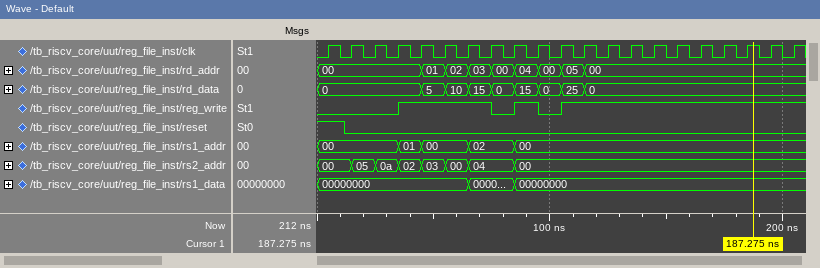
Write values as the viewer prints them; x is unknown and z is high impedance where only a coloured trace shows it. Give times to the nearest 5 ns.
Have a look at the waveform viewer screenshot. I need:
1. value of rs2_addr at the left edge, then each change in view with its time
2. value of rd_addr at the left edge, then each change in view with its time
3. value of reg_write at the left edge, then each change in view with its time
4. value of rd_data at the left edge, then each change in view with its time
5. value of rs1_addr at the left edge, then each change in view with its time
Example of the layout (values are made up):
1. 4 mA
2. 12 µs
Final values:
1. 00, 05 at 15 ns, 0a at 25 ns, 02 at 35 ns, 03 at 45 ns, 00 at 55 ns, 04 at 65 ns, 00 at 85 ns
2. 00, 01 at 45 ns, 02 at 55 ns, 03 at 65 ns, 00 at 75 ns, 04 at 85 ns, 00 at 95 ns, 05 at 105 ns, 00 at 115 ns
3. 0, 1 at 35 ns, 0 at 75 ns, 1 at 85 ns, 0 at 95 ns, 1 at 105 ns
4. 0, 5 at 45 ns, 10 at 55 ns, 15 at 65 ns, 0 at 75 ns, 15 at 85 ns, 0 at 95 ns, 25 at 105 ns, 0 at 115 ns
5. 00, 01 at 35 ns, 00 at 45 ns, 02 at 65 ns, 00 at 85 ns
